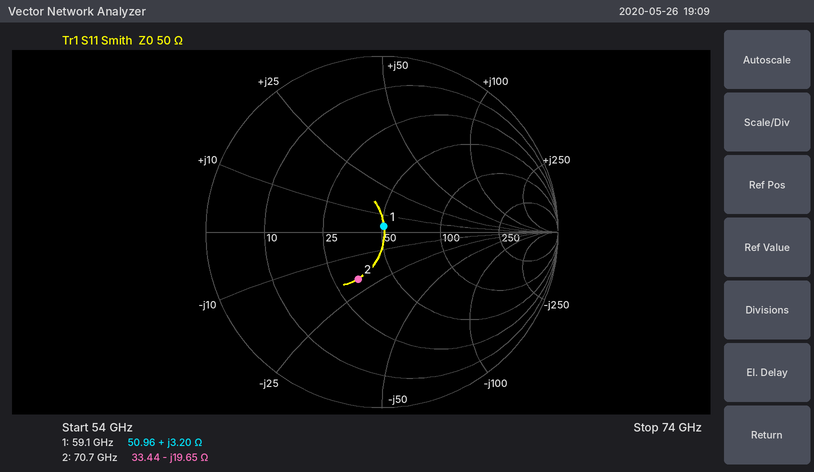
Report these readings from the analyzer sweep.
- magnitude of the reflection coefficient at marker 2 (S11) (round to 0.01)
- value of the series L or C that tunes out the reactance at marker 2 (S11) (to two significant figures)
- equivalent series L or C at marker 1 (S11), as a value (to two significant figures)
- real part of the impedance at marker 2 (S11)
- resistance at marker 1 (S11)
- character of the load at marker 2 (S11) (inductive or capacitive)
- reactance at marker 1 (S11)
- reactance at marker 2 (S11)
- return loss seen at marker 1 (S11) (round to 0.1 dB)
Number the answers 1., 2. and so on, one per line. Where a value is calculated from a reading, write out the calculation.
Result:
1. 0.30
2. L = 19.65 Ω/(2π × 70.7 GHz) ≈ 44 pH
3. L = 3.2 Ω/(2π × 59.1 GHz) ≈ 8.6 pH
4. 33.44 Ω
5. 50.96 Ω
6. capacitive
7. +3.20 Ω
8. -19.65 Ω
9. 29.6 dB
